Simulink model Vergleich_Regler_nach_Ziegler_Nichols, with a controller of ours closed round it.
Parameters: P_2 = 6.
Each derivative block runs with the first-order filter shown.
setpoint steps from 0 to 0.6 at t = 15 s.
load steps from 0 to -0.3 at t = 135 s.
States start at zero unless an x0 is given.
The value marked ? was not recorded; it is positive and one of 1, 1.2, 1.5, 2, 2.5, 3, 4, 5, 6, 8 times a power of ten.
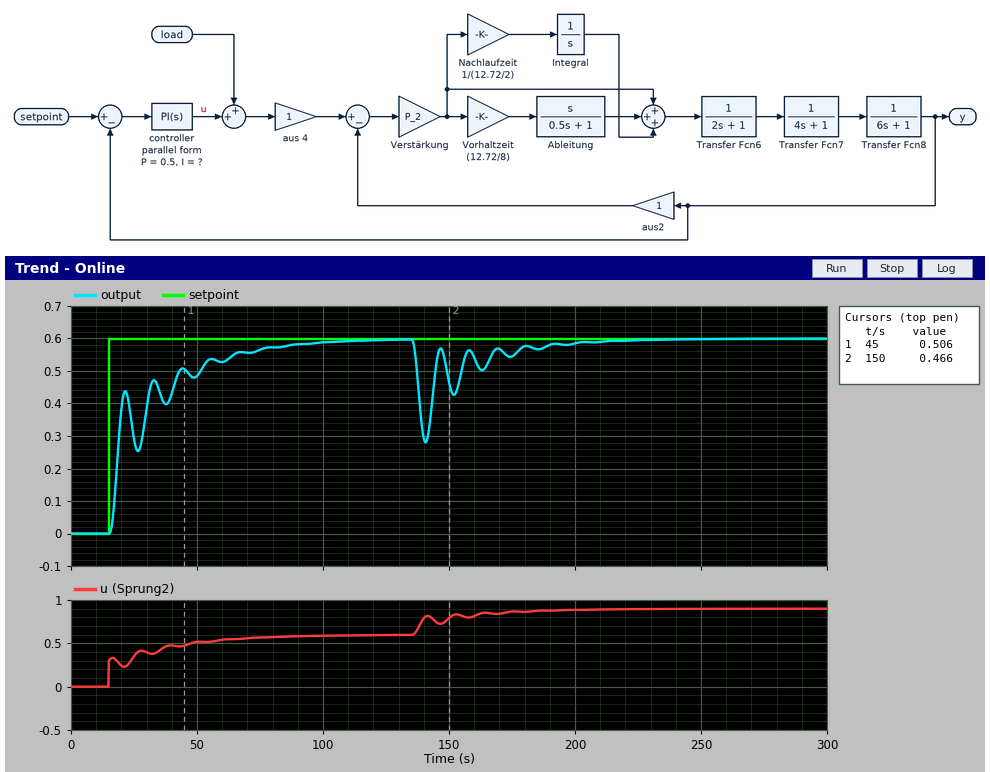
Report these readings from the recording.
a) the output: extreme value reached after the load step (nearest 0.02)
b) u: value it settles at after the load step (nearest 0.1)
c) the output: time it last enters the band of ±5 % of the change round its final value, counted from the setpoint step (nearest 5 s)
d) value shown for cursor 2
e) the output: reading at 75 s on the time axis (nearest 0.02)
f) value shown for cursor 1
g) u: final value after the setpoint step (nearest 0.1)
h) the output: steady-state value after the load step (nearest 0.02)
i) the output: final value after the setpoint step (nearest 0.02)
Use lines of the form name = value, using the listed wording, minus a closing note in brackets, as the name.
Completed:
the output: extreme value reached after the load step = 0.28
u: value it settles at after the load step = 0.9
the output: time it last enters the band of ±5 % of the change round its final value, counted from the setpoint step = 60 s
value shown for cursor 2 = 0.466
the output: reading at 75 s on the time axis = 0.56
value shown for cursor 1 = 0.506
u: final value after the setpoint step = 0.6
the output: steady-state value after the load step = 0.60
the output: final value after the setpoint step = 0.60
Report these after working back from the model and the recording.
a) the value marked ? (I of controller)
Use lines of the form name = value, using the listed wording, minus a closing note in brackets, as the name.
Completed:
the value marked ? = 0.06
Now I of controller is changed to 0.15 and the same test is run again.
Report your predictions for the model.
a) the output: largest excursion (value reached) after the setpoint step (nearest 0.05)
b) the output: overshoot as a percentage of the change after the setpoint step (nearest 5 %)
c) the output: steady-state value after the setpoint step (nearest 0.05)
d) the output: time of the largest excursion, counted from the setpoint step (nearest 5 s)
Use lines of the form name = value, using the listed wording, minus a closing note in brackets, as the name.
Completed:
the output: largest excursion (value reached) after the setpoint step = 0.65
the output: overshoot as a percentage of the change after the setpoint step = 10 %
the output: steady-state value after the setpoint step = 0.60
the output: time of the largest excursion, counted from the setpoint step = 20 s
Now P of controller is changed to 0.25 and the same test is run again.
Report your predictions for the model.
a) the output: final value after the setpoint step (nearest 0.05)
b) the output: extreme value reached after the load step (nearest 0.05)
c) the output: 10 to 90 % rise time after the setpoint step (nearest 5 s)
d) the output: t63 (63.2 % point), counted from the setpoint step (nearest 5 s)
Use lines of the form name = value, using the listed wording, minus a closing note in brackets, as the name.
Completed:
the output: final value after the setpoint step = 0.60
the output: extreme value reached after the load step = 0.25
the output: 10 to 90 % rise time after the setpoint step = 40 s
the output: t63 (63.2 % point), counted from the setpoint step = 15 s
